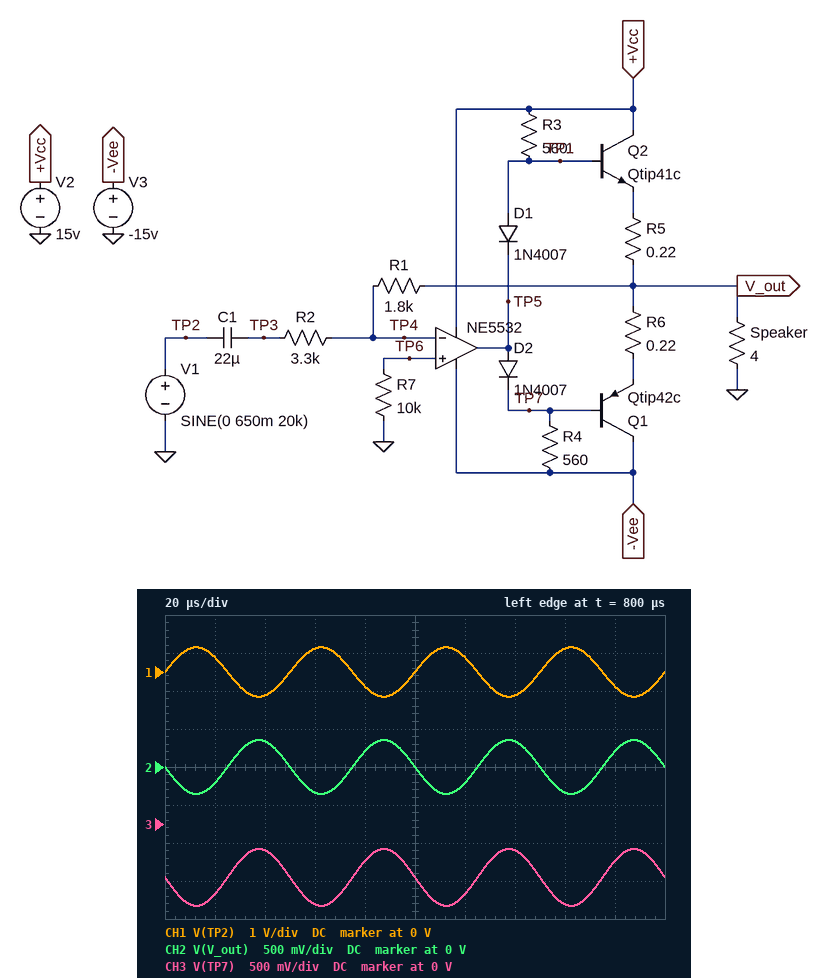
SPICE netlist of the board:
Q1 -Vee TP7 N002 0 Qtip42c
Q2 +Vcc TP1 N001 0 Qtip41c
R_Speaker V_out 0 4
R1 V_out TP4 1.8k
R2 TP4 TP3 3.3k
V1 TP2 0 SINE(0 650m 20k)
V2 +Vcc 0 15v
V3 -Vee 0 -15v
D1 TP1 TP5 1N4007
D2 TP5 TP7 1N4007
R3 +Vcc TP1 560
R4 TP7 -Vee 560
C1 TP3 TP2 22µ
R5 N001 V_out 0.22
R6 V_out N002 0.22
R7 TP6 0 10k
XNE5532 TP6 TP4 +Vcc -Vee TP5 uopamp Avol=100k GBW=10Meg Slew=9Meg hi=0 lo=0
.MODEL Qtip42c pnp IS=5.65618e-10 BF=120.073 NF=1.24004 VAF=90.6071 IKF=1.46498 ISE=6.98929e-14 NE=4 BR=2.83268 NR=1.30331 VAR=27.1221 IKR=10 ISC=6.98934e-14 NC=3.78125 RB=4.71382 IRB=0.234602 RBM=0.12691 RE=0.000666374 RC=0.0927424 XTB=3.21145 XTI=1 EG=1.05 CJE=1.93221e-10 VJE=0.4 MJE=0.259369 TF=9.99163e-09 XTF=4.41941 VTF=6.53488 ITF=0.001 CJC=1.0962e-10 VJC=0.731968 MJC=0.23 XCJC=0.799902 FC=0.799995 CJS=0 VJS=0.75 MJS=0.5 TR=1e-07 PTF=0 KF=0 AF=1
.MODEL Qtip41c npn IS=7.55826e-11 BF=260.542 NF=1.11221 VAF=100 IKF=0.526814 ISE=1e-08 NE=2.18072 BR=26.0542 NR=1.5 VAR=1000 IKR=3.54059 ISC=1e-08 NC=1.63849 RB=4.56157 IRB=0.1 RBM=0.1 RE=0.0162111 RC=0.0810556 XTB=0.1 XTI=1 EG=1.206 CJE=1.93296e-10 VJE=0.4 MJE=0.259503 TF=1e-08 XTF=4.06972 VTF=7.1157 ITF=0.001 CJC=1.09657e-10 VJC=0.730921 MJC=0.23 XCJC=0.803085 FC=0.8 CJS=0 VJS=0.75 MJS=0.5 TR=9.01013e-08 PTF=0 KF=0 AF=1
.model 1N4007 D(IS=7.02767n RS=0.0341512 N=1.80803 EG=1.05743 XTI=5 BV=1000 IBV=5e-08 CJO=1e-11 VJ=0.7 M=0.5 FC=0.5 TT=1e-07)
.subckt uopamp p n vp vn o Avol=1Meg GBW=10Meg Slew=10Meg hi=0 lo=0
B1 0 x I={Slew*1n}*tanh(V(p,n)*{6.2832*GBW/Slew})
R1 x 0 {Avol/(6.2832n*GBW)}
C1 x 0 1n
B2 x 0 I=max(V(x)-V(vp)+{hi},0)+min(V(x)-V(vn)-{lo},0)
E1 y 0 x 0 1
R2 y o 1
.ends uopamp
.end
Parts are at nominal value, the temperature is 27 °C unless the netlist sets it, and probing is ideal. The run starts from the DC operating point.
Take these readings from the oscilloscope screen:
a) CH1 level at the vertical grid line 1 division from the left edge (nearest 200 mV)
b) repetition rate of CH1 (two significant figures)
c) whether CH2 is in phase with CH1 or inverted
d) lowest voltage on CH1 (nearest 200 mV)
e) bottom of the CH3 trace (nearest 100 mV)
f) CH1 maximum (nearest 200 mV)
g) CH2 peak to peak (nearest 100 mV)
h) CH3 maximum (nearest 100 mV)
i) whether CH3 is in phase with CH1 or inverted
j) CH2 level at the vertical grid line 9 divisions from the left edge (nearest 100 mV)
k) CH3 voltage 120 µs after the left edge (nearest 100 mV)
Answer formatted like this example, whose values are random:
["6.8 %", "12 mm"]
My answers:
["400 mV", "20 kHz", "inverted", "-600 mV", "-1.1 V", "600 mV", "700 mV", "-300 mV", "inverted", "200 mV", "-900 mV"]
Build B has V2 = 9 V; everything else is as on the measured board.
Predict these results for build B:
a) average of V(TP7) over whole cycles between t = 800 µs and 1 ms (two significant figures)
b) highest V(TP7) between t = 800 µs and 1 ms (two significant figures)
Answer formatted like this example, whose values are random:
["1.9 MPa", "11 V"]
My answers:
["-690 mV", "-310 mV"]
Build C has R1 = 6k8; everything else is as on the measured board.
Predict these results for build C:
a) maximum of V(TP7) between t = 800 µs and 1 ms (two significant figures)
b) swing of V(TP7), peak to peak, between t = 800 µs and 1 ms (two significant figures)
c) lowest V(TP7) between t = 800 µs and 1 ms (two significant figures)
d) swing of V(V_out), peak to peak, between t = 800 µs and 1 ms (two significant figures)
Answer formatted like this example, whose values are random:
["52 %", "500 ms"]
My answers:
["710 mV", "2.8 V", "-2.1 V", "2.7 V"]
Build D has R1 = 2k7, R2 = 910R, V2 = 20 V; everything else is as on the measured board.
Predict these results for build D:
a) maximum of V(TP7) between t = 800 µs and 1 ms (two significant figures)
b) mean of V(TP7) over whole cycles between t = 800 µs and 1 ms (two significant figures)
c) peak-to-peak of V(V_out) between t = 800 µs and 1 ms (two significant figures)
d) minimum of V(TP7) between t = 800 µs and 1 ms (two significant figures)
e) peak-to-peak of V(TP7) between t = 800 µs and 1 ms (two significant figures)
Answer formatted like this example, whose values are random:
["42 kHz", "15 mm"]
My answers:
["1.3 V", "-710 mV", "3.9 V", "-2.7 V", "4.1 V"]
